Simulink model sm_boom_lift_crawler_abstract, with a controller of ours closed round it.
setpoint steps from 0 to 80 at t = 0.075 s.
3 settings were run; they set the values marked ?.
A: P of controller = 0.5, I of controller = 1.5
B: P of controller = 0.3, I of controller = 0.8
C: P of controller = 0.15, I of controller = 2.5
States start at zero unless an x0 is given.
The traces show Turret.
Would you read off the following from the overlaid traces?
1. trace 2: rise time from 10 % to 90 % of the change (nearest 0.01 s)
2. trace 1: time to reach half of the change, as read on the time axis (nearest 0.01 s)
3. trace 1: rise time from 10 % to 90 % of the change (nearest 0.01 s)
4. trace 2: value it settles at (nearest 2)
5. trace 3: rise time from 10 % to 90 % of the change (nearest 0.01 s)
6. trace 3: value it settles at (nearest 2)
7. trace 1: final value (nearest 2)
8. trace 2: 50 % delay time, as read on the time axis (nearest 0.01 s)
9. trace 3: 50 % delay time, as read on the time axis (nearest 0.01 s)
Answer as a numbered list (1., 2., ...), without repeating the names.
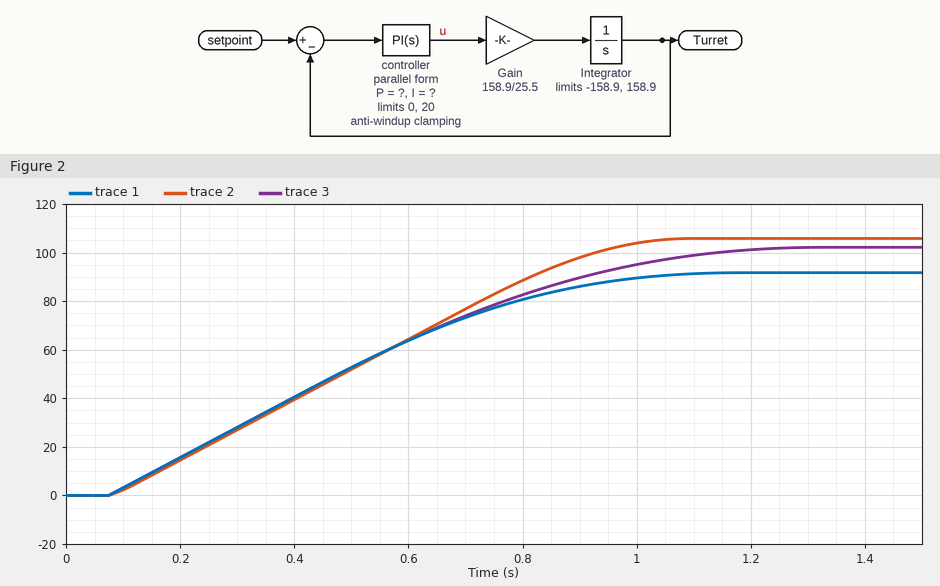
1. 0.70 s
2. 0.44 s
3. 0.68 s
4. 106
5. 0.78 s
6. 102
7. 92
8. 0.51 s
9. 0.49 s
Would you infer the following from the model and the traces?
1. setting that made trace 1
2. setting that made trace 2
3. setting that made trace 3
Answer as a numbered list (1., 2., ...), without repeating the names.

1. A
2. C
3. B
